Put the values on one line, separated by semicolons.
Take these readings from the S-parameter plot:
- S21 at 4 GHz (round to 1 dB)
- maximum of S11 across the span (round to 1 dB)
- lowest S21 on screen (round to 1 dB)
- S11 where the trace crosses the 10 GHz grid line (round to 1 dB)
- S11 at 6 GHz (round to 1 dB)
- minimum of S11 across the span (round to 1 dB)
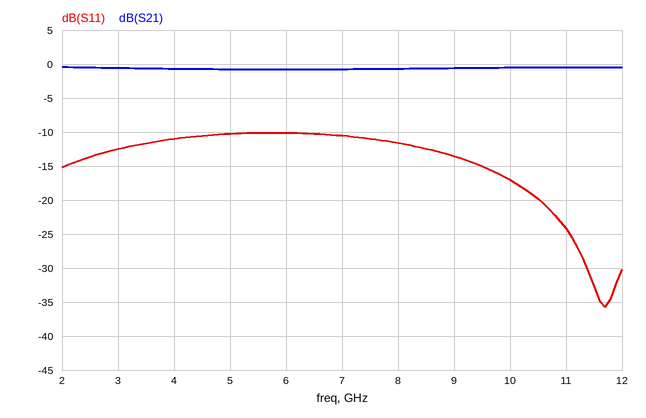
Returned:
-1 dB; -10 dB; -1 dB; -17 dB; -10 dB; -36 dB
